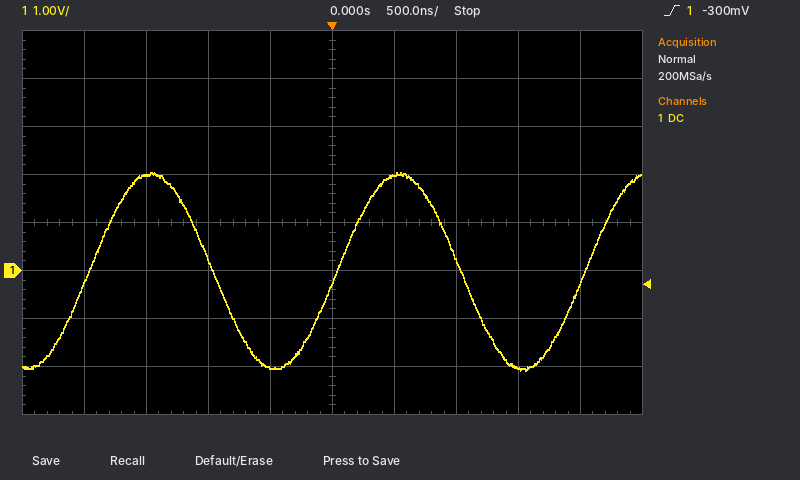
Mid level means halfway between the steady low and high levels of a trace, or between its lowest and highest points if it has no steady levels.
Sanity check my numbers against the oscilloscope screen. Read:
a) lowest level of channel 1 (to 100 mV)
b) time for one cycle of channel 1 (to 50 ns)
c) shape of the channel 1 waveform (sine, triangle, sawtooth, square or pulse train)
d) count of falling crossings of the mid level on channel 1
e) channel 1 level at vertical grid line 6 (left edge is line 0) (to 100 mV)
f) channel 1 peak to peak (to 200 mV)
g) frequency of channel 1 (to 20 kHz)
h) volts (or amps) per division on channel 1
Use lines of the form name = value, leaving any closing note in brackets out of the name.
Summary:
lowest level of channel 1 = -2.1 V
time for one cycle of channel 1 = 2.00 µs
shape of the channel 1 waveform = sine
count of falling crossings of the mid level on channel 1 = 2
channel 1 level at vertical grid line 6 (left edge is line 0) = 2.0 V
channel 1 peak to peak = 4.2 V
frequency of channel 1 = 500 kHz
volts (or amps) per division on channel 1 = 1 V
